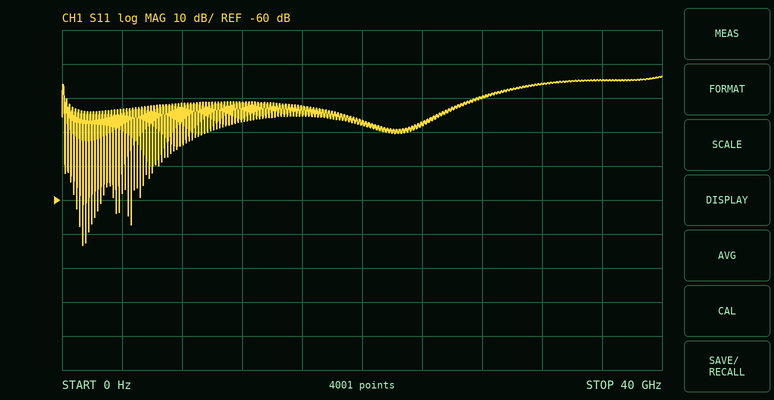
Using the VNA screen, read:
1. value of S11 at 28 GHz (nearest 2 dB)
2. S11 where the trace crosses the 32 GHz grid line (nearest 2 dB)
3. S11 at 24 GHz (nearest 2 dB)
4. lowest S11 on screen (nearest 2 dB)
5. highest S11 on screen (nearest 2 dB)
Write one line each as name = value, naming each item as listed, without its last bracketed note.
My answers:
value of S11 at 28 GHz = -30 dB
S11 where the trace crosses the 32 GHz grid line = -26 dB
S11 at 24 GHz = -38 dB
lowest S11 on screen = -74 dB
highest S11 on screen = -24 dB
